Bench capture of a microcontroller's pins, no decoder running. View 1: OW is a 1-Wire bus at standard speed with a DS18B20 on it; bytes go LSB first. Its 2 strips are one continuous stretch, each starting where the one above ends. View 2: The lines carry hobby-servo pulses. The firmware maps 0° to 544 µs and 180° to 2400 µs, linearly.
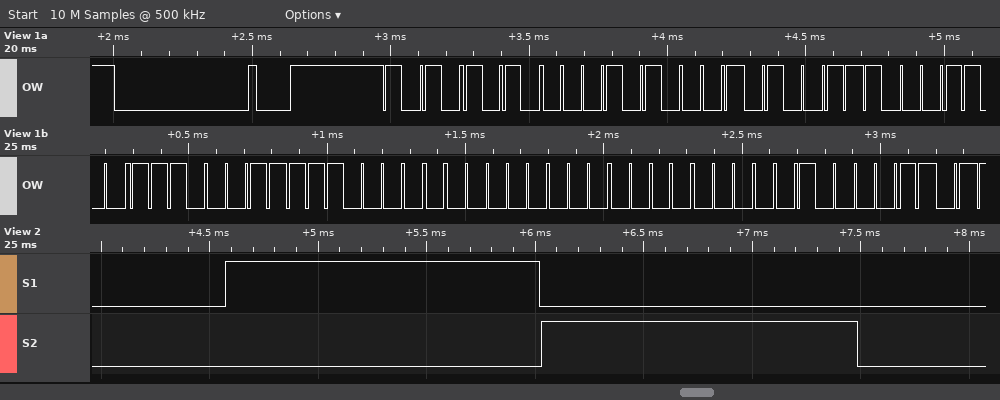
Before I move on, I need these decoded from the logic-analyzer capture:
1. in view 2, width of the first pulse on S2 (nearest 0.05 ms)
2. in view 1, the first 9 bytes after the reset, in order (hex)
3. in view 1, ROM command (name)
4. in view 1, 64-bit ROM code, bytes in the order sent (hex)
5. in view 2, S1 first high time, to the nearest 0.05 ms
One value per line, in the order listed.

1.45 ms
55 28 CA 31 C7 07 00 00 C2
Match ROM
28 CA 31 C7 07 00 00 C2
1.45 ms
